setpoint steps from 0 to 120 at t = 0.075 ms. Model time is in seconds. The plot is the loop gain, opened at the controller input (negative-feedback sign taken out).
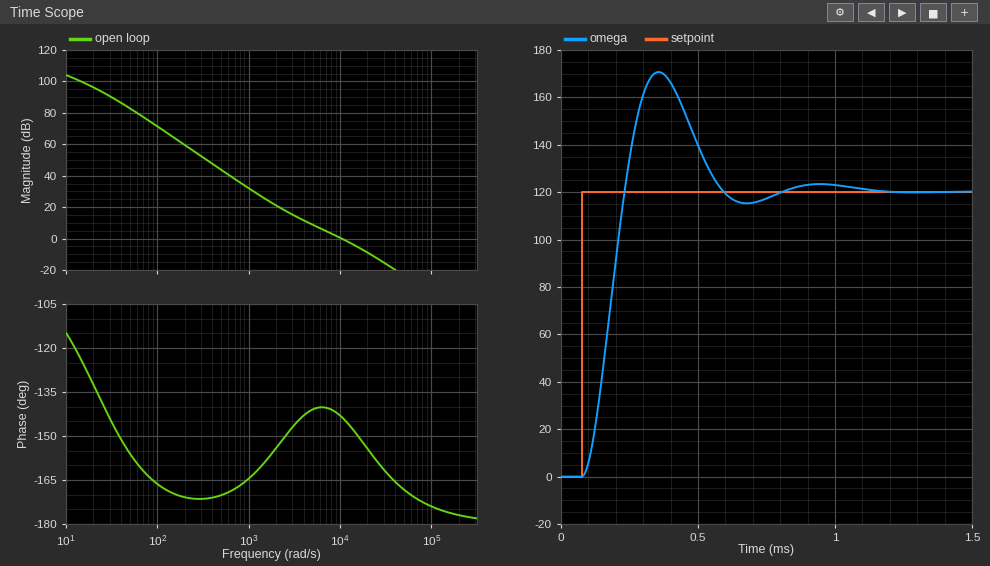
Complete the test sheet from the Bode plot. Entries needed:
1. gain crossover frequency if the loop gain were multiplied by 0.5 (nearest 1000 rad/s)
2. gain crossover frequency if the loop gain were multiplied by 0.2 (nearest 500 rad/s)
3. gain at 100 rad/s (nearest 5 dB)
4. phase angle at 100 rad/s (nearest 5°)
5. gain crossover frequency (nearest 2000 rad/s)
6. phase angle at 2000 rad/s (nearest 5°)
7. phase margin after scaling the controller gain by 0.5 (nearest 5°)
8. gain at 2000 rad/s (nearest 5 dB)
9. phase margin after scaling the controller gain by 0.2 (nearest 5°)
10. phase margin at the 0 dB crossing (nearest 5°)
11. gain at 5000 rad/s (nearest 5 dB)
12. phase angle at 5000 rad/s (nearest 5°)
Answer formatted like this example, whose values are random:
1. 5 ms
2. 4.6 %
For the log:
1. 6000 rad/s
2. 3500 rad/s
3. 70 dB
4. -165°
5. 10000 rad/s
6. -155°
7. 40°
8. 20 dB
9. 35°
10. 35°
11. 10 dB
12. -140°
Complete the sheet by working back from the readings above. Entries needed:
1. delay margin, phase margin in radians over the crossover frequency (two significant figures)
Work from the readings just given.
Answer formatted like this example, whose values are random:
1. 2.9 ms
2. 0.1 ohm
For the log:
1. 0.000061 s
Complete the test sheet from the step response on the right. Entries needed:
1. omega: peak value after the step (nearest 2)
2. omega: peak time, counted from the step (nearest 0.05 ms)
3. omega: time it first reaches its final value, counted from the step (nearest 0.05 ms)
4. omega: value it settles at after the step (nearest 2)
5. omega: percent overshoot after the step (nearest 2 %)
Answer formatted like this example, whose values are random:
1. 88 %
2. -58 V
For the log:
1. 170
2. 0.30 ms
3. 0.15 ms
4. 120
5. 42 %
